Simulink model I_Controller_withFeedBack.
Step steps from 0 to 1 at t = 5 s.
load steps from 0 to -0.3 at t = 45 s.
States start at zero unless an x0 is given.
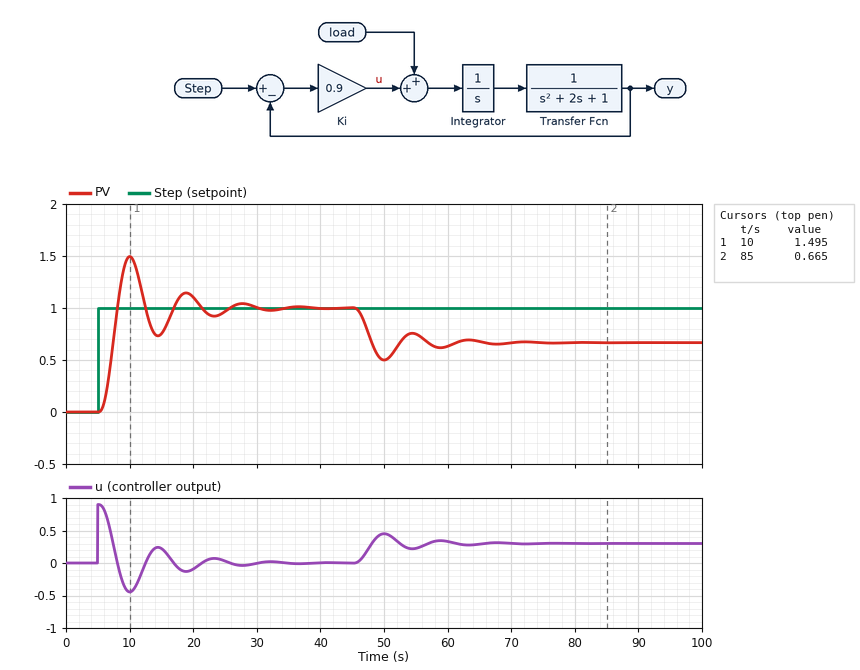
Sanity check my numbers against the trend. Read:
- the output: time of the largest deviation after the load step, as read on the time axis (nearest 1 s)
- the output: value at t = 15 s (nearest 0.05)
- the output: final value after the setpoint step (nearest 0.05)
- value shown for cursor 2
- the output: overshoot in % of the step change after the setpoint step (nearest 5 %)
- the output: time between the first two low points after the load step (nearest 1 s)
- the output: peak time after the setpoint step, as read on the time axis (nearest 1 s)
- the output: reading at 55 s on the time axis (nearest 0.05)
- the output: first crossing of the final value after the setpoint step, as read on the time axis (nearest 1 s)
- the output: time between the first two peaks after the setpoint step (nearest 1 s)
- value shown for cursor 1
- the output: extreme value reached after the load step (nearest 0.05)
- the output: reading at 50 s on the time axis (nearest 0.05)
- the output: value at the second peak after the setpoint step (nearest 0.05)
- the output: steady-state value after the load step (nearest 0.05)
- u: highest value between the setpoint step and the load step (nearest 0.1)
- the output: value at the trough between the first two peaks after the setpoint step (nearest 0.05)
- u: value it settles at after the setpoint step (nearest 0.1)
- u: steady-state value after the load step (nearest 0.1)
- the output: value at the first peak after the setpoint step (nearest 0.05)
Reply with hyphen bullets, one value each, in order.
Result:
- 50 s
- 0.75
- 1.00
- 0.665
- 50 %
- 9 s
- 10 s
- 0.75
- 8 s
- 9 s
- 1.495
- 0.50
- 0.50
- 1.15
- 0.65
- 0.9
- 0.75
- 0.0
- 0.3
- 1.50
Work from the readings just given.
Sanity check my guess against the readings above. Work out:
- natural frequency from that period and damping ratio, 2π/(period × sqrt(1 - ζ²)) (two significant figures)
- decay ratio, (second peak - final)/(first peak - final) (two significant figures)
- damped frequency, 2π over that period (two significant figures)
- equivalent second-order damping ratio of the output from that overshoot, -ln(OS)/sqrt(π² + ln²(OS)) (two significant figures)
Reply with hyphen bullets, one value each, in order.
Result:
- 0.72 rad/s
- 0.30
- 0.70 rad/s
- 0.22
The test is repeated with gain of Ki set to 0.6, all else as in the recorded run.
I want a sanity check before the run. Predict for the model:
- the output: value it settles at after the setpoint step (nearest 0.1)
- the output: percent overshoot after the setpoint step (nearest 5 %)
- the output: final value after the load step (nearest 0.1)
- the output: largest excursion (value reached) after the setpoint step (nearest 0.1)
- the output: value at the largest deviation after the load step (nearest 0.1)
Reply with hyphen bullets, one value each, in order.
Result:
- 1.0
- 30 %
- 0.5
- 1.3
- 0.3
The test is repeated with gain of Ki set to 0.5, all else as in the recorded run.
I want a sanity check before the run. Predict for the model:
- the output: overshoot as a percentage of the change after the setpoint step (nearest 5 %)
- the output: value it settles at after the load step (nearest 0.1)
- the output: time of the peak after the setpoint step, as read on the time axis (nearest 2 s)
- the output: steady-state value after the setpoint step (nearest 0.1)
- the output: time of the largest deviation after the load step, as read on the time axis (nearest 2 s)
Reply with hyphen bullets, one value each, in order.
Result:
- 25 %
- 0.4
- 12 s
- 1.0
- 52 s
